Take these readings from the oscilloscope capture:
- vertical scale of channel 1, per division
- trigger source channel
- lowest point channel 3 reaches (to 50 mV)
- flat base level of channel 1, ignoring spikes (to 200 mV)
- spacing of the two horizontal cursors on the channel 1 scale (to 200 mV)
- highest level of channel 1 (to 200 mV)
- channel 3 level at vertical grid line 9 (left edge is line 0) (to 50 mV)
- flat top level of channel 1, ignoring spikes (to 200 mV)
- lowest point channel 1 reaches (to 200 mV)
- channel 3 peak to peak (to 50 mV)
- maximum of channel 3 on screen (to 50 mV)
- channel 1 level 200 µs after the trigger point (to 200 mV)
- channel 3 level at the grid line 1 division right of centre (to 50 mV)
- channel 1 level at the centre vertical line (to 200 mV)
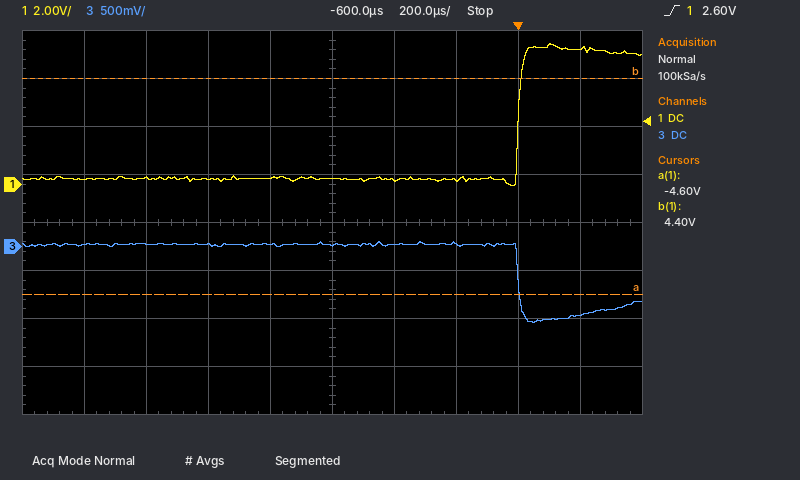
2 V
channel 1
-800 mV
200 mV
9.0 V
5.8 V
-700 mV
5.6 V
0.0 V
850 mV
50 mV
5.6 V
0 mV
200 mV
